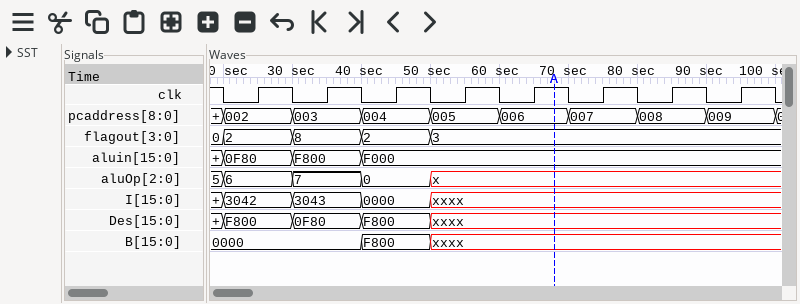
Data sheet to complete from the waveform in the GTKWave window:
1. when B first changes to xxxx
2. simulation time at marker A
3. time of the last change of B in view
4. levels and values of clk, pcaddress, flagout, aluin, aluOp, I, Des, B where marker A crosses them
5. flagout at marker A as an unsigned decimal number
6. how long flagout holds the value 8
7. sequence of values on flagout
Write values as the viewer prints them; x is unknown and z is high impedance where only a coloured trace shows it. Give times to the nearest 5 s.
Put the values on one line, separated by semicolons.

50 s; 70 s; 50 s; clk=1, pcaddress=006, flagout=3, aluin=F000, aluOp=x, I=xxxx, Des=xxxx, B=xxxx; 3; 10 s; 0, 2, 8, 2, 3
